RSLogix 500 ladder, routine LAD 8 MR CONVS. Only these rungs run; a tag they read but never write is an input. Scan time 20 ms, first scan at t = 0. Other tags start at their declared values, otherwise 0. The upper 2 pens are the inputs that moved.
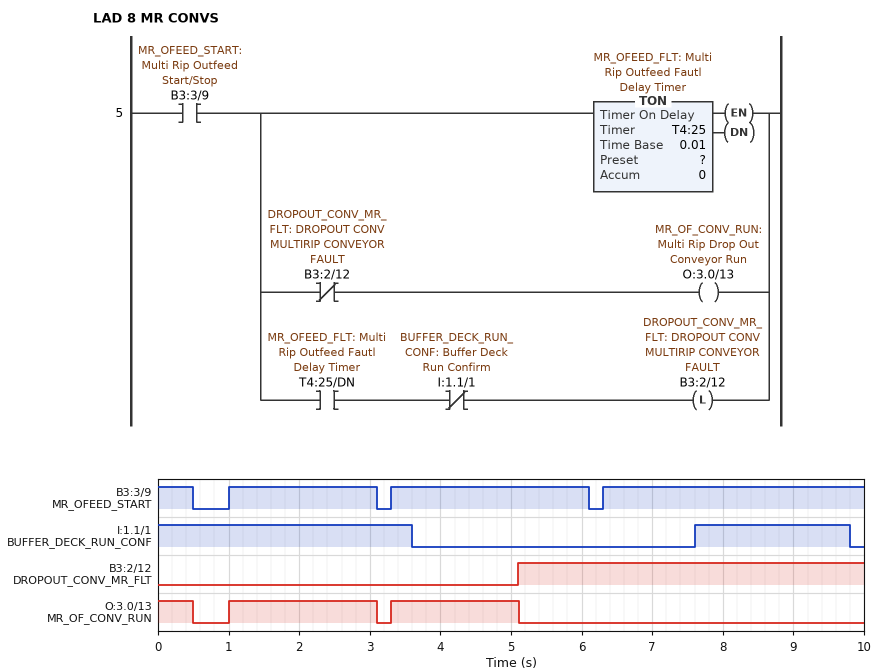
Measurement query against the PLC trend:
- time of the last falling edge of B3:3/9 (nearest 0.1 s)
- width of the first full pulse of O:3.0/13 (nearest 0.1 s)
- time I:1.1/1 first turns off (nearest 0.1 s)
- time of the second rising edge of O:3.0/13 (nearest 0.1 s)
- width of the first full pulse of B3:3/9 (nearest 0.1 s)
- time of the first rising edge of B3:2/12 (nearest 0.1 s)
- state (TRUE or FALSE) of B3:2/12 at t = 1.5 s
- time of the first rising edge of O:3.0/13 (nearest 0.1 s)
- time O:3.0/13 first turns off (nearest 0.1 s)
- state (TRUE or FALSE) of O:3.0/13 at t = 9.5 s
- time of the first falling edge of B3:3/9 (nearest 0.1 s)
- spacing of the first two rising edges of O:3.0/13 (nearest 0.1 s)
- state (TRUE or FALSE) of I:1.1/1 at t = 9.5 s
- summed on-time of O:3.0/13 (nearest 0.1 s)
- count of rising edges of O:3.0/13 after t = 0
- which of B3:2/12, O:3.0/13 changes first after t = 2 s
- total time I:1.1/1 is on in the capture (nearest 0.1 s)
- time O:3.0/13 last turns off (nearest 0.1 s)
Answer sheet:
6.1 s
2.1 s
3.6 s
3.3 s
2.1 s
5.1 s
FALSE
1.0 s
0.5 s
FALSE
0.5 s
2.3 s
TRUE
4.4 s
2
O:3.0/13
5.8 s
5.1 s
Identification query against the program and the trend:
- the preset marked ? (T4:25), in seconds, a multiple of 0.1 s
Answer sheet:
1.8 s
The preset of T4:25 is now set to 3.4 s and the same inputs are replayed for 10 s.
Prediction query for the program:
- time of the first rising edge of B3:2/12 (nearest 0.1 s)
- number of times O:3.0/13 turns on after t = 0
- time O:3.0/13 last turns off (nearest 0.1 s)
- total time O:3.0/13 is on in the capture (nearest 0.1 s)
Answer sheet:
9.8 s
3
9.8 s
8.9 s
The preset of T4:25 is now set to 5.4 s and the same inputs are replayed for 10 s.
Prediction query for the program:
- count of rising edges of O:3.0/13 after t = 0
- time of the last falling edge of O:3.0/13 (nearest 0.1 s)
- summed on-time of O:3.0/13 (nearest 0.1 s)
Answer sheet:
3
6.1 s
9.1 s
